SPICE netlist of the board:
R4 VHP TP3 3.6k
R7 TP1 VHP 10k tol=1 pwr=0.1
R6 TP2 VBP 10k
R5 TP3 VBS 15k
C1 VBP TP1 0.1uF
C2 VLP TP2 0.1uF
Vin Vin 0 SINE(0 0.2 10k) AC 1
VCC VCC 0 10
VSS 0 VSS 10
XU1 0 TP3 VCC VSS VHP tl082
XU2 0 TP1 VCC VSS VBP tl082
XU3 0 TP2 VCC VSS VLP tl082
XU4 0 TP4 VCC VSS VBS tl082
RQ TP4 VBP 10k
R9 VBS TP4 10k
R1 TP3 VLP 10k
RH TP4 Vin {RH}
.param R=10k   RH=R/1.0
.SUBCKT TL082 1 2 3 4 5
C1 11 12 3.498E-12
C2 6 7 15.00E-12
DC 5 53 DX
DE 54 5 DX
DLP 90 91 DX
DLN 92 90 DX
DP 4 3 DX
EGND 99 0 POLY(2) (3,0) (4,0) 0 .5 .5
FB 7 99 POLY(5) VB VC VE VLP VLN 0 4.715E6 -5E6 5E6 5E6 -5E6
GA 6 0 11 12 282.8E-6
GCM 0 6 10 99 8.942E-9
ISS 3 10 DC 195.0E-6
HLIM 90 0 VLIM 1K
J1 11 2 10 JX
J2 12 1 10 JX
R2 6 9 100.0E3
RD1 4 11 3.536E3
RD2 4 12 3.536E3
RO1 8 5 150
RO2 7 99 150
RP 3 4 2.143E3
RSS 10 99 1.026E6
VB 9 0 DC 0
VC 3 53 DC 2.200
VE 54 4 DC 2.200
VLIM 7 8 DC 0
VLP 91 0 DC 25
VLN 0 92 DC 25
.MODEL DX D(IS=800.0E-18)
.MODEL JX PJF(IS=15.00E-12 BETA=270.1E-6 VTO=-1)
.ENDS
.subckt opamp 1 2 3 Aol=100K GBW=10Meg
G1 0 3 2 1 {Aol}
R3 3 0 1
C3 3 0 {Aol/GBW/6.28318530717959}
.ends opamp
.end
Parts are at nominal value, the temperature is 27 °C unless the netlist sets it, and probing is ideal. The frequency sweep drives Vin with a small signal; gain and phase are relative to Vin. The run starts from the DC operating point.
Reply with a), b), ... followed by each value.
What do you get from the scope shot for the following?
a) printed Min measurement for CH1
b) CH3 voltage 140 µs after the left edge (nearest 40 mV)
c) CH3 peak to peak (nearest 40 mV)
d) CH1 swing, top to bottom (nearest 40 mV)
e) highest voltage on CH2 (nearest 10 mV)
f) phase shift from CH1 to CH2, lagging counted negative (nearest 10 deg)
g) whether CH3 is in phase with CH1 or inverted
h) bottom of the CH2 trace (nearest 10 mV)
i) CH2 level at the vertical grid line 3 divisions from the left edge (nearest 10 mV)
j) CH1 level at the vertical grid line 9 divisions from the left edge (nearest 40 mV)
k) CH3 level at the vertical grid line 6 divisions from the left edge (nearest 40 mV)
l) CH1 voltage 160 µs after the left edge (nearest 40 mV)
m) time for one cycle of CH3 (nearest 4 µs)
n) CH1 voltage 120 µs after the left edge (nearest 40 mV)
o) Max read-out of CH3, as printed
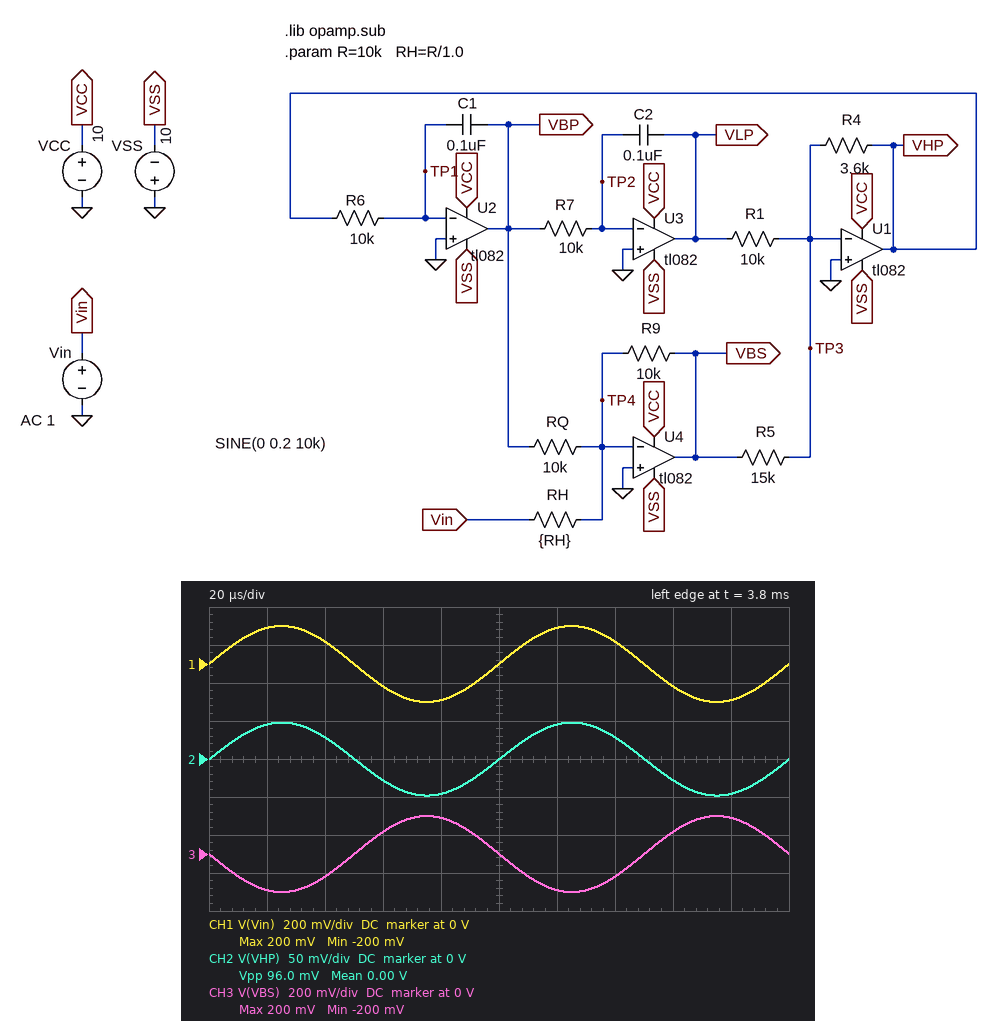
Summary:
a) -200 mV
b) -120 mV
c) 400 mV
d) 400 mV
e) 50 mV
f) 0 deg
g) inverted
h) -50 mV
i) -30 mV
j) -200 mV
k) -200 mV
l) -120 mV
m) 100 µs
n) 200 mV
o) 200 mV
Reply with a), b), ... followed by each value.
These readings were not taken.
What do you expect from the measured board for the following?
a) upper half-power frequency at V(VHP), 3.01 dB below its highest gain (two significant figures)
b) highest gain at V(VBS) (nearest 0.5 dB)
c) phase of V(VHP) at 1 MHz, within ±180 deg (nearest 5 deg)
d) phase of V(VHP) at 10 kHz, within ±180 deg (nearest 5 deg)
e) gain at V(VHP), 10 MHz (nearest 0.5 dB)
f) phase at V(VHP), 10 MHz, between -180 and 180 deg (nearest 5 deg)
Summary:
a) 130 Hz
b) 0 dB
c) -75 deg
d) 0 deg
e) -52.0 dB
f) 60 deg
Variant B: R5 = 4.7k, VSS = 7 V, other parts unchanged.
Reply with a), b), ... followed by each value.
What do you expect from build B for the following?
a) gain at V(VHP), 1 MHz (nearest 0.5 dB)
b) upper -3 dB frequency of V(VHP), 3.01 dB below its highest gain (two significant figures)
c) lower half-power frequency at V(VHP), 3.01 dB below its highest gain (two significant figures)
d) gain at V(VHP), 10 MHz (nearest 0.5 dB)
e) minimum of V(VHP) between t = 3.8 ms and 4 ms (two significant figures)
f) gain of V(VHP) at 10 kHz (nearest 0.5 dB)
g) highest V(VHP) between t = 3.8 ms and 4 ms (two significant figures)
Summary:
a) -5.0 dB
b) 1.0 MHz
c) 88 Hz
d) -44.5 dB
e) -150 mV
f) -2.5 dB
g) 150 mV
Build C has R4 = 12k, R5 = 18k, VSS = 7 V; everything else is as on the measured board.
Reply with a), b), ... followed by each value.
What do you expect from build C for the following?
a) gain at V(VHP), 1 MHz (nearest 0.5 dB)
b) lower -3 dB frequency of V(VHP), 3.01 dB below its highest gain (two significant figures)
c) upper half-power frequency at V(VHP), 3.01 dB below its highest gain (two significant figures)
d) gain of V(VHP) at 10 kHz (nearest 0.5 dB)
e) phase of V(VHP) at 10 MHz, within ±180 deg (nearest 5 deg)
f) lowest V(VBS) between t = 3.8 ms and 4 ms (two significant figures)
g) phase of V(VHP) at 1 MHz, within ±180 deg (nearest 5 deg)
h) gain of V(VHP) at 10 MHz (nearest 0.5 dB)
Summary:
a) -7.0 dB
b) 150 Hz
c) 360 Hz
d) -3.5 dB
e) 65 deg
f) -200 mV
g) -90 deg
h) -49.5 dB
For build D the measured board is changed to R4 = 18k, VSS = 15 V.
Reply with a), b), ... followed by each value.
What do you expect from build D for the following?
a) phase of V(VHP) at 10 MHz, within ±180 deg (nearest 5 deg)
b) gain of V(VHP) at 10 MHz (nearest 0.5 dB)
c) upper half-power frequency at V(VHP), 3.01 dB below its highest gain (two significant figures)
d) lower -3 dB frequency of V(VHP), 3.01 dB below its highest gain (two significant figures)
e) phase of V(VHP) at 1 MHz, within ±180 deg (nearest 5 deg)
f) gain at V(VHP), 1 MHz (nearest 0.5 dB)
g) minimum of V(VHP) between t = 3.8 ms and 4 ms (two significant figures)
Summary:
a) 65 deg
b) -47.5 dB
c) 410 kHz
d) 180 Hz
e) -100 deg
f) -3.5 dB
g) -240 mV
